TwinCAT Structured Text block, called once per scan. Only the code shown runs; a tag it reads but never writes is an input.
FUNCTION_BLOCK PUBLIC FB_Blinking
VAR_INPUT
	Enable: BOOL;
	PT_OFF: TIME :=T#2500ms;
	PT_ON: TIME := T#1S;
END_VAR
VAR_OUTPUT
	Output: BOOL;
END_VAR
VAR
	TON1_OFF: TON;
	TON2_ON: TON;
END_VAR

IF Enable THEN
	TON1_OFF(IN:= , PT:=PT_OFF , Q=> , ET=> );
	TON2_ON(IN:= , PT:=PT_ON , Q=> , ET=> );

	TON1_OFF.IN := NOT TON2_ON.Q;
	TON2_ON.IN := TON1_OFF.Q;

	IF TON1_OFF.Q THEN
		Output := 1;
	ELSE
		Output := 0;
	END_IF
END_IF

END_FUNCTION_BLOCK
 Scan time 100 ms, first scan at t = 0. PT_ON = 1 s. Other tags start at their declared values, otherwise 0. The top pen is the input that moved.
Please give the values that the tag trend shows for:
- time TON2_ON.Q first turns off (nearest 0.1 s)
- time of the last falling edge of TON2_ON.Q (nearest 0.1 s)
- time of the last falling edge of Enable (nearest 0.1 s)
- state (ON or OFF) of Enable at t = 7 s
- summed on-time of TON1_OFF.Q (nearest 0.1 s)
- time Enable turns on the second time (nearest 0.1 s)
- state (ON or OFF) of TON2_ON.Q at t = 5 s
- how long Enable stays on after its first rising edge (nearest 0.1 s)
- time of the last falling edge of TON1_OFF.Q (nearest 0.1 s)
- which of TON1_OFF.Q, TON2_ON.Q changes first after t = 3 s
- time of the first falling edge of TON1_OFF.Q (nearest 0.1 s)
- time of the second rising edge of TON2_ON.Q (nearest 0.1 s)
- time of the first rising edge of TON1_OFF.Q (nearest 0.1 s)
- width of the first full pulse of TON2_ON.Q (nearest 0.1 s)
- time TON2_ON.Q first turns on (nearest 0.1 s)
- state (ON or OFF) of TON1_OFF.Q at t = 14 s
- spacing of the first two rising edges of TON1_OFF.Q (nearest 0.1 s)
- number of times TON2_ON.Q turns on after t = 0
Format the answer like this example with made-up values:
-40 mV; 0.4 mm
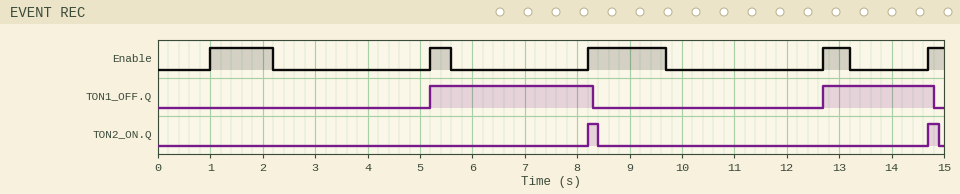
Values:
8.4 s; 14.9 s; 13.2 s; OFF; 5.2 s; 5.2 s; OFF; 1.2 s; 14.8 s; TON1_OFF.Q; 8.3 s; 14.7 s; 5.2 s; 0.2 s; 8.2 s; ON; 7.5 s; 2
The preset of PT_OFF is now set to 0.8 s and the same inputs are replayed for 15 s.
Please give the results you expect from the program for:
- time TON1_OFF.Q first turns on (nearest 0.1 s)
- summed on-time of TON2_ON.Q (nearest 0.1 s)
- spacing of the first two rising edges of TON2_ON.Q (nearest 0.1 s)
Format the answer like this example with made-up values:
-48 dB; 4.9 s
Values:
1.9 s; 0.6 s; 4.1 s
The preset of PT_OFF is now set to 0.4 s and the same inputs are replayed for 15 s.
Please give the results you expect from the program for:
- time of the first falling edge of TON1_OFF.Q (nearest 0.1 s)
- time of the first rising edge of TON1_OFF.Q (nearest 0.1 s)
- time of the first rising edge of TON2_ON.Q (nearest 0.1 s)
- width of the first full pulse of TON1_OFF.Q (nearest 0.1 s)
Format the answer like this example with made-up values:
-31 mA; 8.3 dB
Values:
5.3 s; 1.5 s; 5.2 s; 3.8 s
